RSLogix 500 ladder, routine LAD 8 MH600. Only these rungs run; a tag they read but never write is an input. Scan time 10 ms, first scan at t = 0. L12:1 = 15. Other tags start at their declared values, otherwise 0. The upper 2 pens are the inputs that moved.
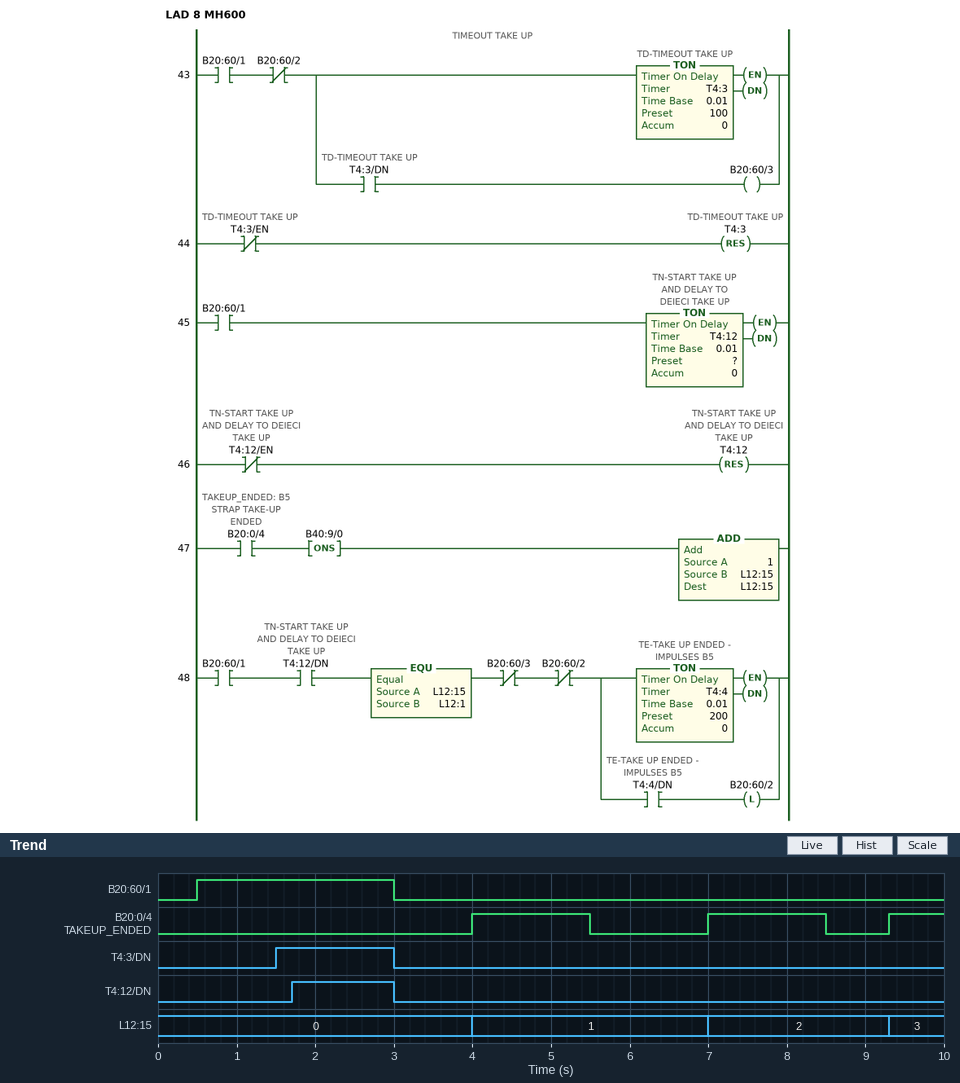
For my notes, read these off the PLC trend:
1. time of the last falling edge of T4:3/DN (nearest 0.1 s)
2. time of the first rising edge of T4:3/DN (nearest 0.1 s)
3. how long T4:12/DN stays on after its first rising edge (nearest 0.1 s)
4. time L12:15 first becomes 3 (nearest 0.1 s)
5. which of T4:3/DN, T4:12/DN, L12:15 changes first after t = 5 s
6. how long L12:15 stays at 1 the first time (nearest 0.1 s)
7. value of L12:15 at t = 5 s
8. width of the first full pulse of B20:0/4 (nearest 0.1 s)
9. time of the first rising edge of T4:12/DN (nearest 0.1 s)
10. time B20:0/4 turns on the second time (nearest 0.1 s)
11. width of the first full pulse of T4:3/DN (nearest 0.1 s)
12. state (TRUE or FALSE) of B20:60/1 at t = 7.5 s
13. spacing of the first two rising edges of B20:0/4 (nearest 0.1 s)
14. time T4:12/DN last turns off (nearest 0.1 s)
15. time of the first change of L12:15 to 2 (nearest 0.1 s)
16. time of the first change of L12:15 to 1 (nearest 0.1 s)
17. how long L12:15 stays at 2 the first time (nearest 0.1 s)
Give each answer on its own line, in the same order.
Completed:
3.0 s
1.5 s
1.3 s
9.3 s
L12:15
3.0 s
1
1.5 s
1.7 s
7.0 s
1.5 s
FALSE
3.0 s
3.0 s
7.0 s
4.0 s
2.3 s
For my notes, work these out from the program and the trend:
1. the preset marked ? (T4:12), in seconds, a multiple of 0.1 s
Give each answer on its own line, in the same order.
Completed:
1.2 s
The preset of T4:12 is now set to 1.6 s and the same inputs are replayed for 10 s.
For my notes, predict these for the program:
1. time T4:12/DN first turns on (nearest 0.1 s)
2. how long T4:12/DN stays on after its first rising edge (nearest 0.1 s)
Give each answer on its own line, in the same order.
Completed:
2.1 s
0.9 s
